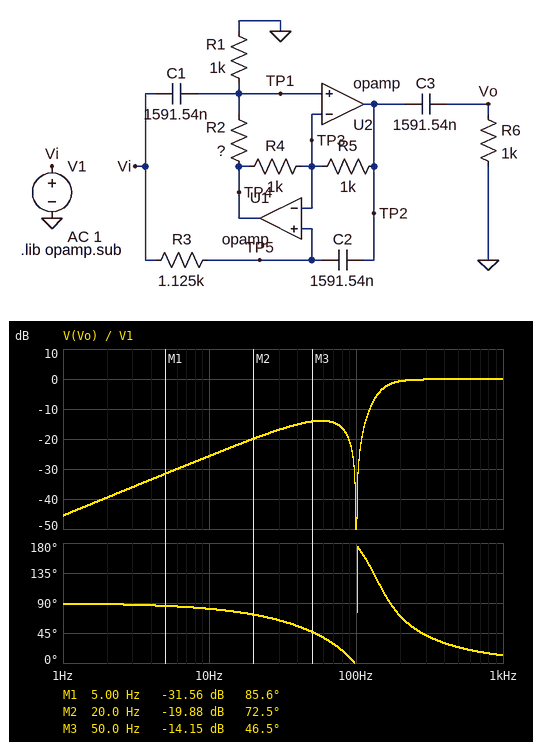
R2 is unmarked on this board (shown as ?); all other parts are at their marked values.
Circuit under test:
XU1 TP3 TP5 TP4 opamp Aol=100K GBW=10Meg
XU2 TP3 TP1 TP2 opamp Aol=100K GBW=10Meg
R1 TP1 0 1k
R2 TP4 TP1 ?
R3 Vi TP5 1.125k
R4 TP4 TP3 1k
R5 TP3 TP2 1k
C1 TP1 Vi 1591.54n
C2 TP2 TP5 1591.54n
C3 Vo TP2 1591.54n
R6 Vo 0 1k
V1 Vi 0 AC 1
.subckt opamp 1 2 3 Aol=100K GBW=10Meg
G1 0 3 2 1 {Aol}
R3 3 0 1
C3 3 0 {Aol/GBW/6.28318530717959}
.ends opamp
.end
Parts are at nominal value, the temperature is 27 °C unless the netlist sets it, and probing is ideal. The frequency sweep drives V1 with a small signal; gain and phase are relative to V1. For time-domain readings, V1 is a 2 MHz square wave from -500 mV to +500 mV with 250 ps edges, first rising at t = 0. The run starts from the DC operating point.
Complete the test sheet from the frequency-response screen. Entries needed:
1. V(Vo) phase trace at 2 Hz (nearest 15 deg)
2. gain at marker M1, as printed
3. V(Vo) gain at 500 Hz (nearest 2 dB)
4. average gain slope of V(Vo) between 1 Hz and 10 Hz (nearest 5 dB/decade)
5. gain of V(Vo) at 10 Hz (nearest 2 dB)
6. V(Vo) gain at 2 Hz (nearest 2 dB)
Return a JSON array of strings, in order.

["90 deg", "-31.56 dB", "0 dB", "20 dB/decade", "-26 dB", "-40 dB"]
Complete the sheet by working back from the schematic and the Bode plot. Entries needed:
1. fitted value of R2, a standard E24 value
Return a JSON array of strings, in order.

["470 Ω"]
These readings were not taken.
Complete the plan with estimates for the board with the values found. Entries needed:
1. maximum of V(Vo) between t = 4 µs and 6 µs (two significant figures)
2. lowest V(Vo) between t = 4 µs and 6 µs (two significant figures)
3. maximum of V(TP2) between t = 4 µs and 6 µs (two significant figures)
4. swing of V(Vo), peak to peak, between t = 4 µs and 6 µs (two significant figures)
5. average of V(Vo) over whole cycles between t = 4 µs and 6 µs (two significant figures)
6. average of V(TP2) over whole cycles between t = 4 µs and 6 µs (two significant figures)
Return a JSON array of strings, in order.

["1.2 V", "-210 mV", "940 mV", "1.4 V", "500 mV", "230 mV"]
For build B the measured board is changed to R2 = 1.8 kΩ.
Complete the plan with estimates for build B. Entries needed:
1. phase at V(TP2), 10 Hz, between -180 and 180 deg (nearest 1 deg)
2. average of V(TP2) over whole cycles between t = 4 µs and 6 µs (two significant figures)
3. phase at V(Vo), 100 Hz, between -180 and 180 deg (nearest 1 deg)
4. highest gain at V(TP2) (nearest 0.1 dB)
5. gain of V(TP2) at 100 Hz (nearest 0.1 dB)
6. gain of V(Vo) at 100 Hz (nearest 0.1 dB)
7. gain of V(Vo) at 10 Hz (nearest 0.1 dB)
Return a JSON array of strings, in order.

["168 deg", "900 mV", "108 deg", "2.1 dB", "1.9 dB", "-1.1 dB", "-21.8 dB"]
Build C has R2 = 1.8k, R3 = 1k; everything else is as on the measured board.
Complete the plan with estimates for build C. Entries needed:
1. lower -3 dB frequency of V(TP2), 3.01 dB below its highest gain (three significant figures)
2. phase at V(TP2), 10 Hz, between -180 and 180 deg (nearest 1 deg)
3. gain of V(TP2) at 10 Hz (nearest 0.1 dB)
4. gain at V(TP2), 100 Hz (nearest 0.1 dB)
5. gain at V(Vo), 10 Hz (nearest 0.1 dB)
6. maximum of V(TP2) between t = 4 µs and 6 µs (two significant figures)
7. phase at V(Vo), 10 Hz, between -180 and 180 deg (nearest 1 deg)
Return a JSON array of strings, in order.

["28.9 Hz", "170 deg", "-1.7 dB", "2.4 dB", "-21.8 dB", "1.6 V", "-106 deg"]
